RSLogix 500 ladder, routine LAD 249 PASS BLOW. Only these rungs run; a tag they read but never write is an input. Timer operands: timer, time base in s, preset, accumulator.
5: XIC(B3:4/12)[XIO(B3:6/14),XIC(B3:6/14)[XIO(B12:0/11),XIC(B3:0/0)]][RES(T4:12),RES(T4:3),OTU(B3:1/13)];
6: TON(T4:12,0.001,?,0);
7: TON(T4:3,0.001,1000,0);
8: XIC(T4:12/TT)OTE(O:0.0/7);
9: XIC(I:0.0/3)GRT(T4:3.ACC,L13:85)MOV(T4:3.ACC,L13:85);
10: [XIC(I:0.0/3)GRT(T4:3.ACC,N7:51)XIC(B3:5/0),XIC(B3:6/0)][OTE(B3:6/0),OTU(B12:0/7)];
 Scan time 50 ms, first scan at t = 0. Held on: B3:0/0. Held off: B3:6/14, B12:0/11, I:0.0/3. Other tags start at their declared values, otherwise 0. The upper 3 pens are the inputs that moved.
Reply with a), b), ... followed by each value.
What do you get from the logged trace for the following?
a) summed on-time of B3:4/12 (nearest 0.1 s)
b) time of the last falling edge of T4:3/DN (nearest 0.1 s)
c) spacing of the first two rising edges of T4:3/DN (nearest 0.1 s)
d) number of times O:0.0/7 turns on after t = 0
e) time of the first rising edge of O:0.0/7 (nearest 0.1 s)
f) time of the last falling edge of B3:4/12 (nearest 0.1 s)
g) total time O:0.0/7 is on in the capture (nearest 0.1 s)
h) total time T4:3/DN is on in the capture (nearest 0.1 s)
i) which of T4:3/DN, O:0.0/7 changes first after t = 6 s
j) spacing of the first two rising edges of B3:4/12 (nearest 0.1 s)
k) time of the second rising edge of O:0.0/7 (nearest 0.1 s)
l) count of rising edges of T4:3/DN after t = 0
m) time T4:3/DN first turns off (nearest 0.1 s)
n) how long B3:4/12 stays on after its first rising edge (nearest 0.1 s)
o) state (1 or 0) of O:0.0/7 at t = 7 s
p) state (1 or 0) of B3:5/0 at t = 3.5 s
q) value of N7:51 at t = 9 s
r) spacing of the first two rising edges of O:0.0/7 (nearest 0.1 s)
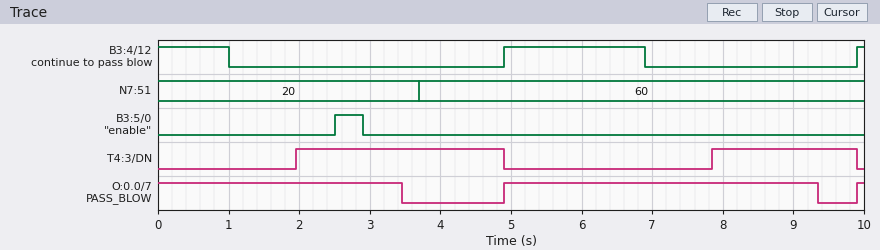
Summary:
a) 3.1 s
b) 9.9 s
c) 5.9 s
d) 2
e) 4.9 s
f) 6.9 s
g) 8.0 s
h) 5.0 s
i) T4:3/DN
j) 5.0 s
k) 9.9 s
l) 2
m) 4.9 s
n) 2.0 s
o) 1
p) 0
q) 60
r) 5.0 s
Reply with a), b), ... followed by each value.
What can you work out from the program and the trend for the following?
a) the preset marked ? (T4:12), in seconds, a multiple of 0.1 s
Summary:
a) 2.5 s
